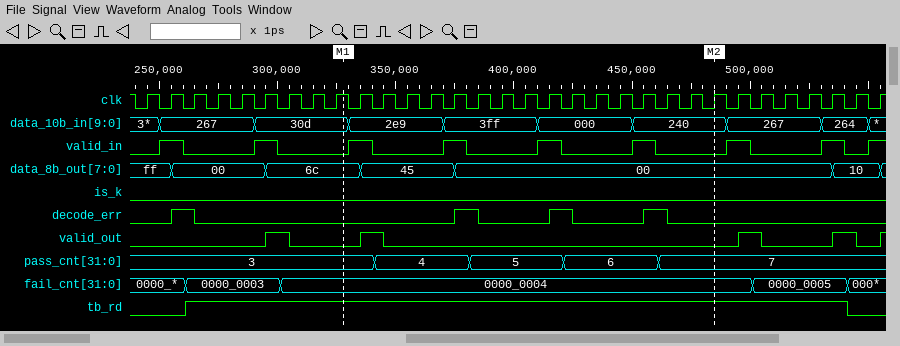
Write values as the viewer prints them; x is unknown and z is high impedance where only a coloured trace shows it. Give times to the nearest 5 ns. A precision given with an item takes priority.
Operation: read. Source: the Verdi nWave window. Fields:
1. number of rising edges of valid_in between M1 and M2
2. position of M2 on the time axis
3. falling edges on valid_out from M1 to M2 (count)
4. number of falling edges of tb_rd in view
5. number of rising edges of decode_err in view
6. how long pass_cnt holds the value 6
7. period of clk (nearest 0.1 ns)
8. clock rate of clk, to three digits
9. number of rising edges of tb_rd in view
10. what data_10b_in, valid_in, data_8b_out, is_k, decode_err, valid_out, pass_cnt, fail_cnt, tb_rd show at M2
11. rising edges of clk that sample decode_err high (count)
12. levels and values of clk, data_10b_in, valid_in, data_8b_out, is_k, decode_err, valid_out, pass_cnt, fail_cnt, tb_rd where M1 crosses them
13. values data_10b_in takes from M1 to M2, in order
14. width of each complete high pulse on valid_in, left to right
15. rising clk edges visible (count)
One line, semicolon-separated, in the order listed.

4; 485 ns; 1; 1; 4; 40 ns; 10 ns; 100 MHz; 1; data_10b_in=240, valid_in=0, data_8b_out=00, is_k=0, decode_err=0, valid_out=0, pass_cnt=7, fail_cnt=0000_0004, tb_rd=1; 4; clk=1, data_10b_in=30d, valid_in=0, data_8b_out=6c, is_k=0, decode_err=0, valid_out=0, pass_cnt=3, fail_cnt=0000_0004, tb_rd=1; 30d, 2e9, 3ff, 000, 240; 10 ns, 10 ns, 10 ns, 10 ns, 10 ns, 10 ns, 10 ns, 10 ns; 32
